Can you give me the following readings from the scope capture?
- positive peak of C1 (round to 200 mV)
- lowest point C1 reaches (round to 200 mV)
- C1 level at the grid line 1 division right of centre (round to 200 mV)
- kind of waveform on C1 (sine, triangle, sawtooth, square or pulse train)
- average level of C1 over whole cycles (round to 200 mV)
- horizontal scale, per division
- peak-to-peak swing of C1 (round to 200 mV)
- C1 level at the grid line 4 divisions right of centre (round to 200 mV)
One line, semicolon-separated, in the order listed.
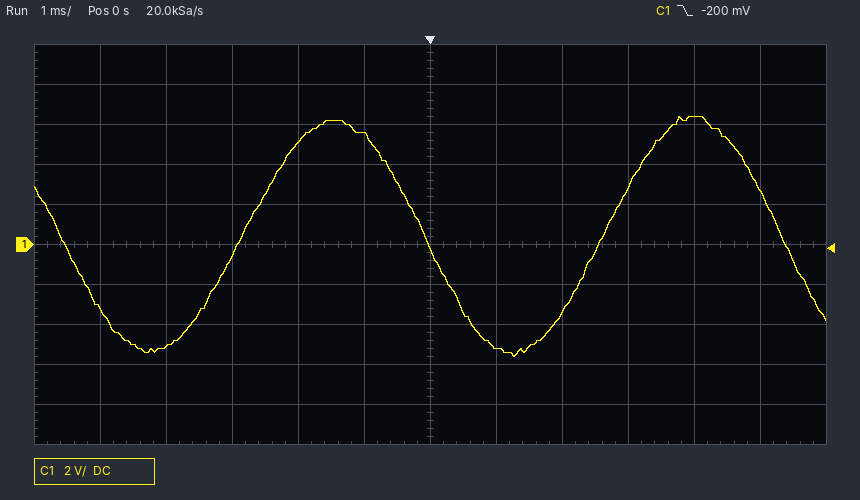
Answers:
6.4 V; -5.6 V; -5.2 V; sine; 400 mV; 1 ms; 12.0 V; 6.4 V
